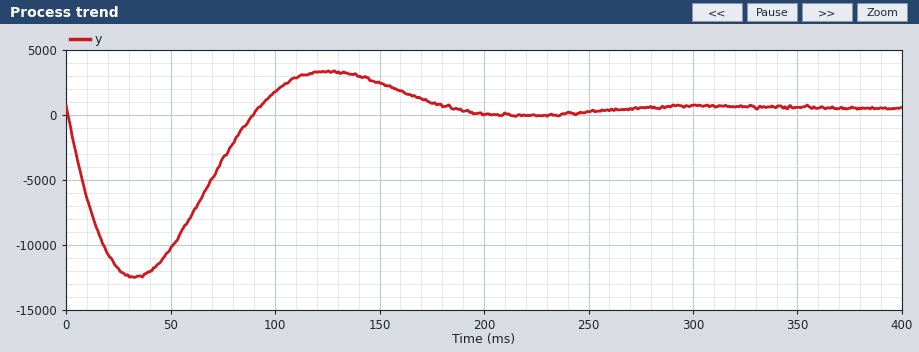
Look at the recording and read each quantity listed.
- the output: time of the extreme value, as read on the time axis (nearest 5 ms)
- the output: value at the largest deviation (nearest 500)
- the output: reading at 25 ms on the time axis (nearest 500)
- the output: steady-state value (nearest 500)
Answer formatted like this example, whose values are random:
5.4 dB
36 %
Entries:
35 ms
-12500
-12000
500
